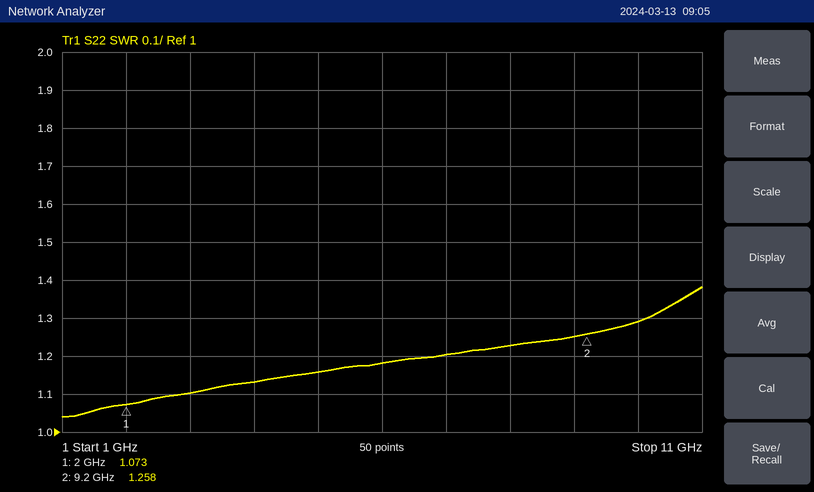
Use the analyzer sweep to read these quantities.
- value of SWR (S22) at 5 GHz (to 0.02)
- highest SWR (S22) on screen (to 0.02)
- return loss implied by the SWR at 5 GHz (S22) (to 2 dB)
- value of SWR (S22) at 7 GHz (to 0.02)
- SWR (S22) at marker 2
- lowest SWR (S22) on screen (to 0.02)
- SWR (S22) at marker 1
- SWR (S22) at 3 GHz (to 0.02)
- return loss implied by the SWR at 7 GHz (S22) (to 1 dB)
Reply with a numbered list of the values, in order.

1. 1.16
2. 1.38
3. 22 dB
4. 1.20
5. 1.258
6. 1.04
7. 1.073
8. 1.10
9. 21 dB
